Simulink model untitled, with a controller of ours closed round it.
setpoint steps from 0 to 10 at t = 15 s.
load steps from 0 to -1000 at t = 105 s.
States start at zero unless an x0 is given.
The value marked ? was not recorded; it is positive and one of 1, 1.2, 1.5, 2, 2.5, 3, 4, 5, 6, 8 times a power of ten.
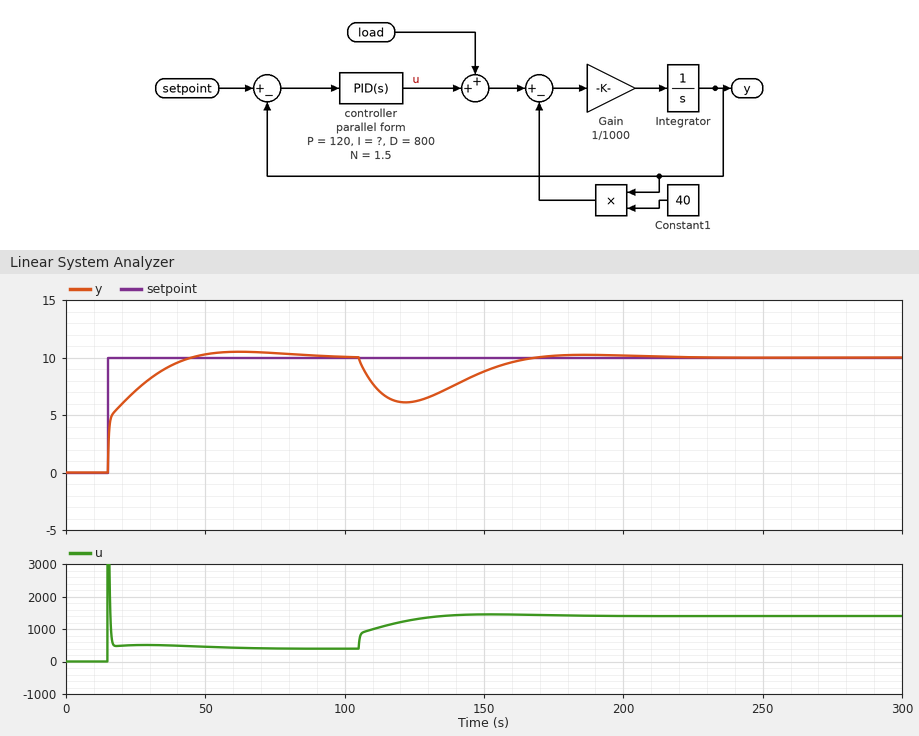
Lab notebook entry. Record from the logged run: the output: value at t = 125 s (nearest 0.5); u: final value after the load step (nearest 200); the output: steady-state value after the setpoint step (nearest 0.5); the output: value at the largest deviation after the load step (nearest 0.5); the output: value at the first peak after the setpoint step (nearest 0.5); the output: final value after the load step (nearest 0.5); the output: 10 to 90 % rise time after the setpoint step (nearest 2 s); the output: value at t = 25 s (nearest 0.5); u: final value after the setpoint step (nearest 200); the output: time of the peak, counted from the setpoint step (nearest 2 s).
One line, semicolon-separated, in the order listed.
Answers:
6.0; 1400; 10.0; 6.0; 10.5; 10.0; 20 s; 7.0; 400; 48 s
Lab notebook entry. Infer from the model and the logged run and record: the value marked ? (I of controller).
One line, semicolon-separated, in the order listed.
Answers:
8
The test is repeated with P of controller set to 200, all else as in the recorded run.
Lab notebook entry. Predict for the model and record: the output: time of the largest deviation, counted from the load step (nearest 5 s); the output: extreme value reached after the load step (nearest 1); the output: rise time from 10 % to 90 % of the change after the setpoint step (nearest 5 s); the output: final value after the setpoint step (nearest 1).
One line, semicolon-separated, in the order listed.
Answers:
15 s; 7; 15 s; 10
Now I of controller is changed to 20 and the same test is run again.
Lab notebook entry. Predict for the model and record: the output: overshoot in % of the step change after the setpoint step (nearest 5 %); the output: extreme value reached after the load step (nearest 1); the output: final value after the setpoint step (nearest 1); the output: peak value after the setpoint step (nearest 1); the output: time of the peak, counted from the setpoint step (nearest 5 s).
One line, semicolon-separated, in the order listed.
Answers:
15 %; 7; 10; 11; 30 s
